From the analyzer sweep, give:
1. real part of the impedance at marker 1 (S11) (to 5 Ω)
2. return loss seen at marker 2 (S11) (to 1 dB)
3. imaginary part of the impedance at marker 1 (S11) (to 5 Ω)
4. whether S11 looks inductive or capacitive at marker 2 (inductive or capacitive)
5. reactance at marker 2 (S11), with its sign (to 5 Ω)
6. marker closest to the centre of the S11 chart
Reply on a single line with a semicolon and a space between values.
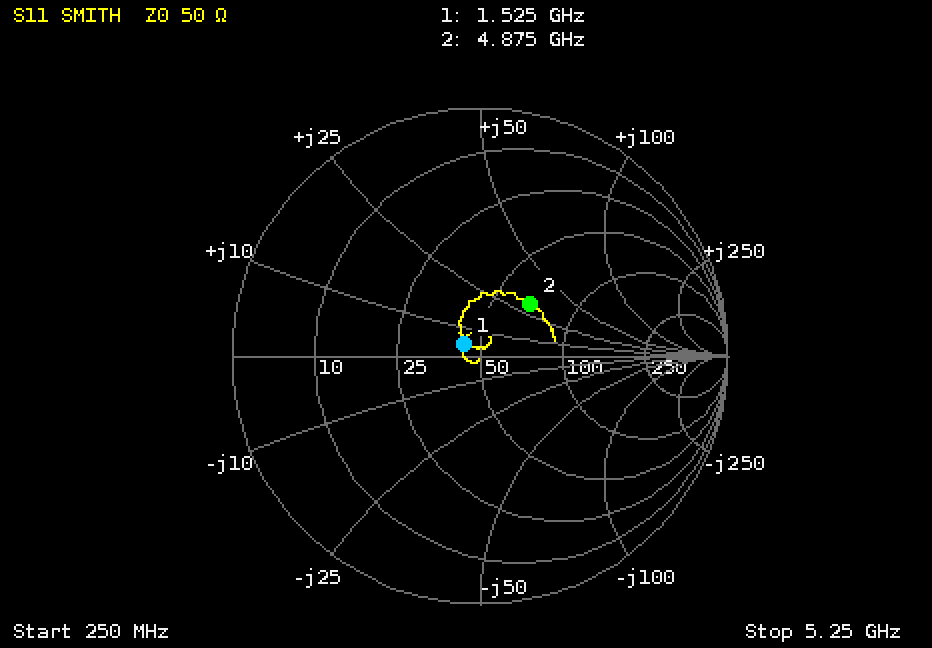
45 Ω; 11 dB; +5 Ω; inductive; +30 Ω; marker 1
